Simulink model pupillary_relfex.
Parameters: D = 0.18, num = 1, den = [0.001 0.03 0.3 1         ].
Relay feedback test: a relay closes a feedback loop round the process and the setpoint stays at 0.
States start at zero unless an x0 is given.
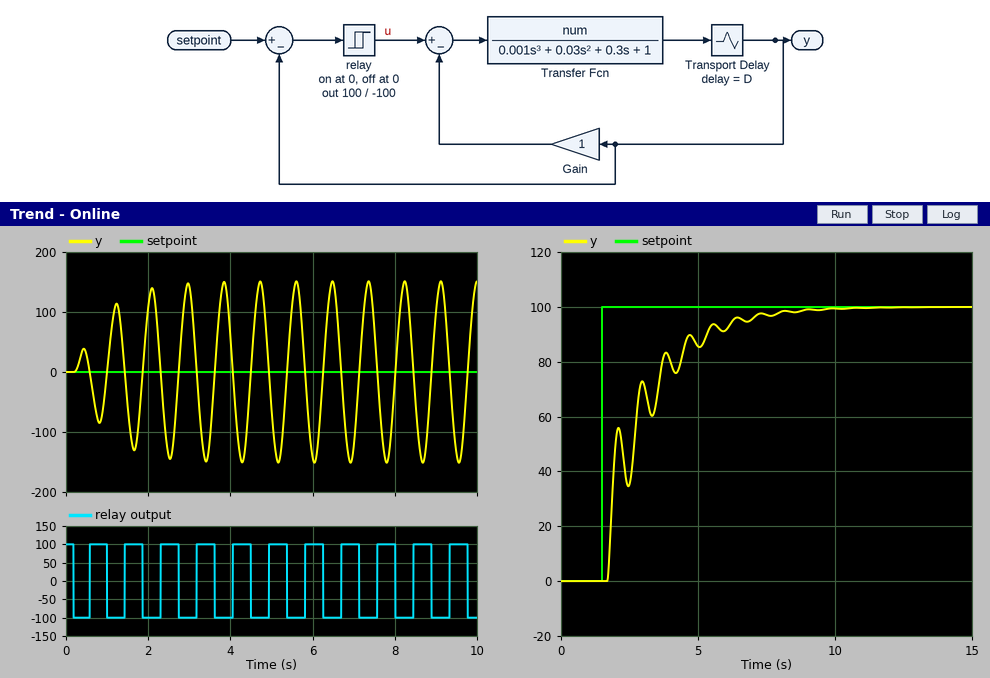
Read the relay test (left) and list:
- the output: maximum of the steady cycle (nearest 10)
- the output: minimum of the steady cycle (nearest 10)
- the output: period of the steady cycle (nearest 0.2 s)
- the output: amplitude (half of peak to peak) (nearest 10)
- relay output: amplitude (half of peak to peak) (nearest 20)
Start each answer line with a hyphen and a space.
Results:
- 150
- -150
- 0.8 s
- 150
- 100
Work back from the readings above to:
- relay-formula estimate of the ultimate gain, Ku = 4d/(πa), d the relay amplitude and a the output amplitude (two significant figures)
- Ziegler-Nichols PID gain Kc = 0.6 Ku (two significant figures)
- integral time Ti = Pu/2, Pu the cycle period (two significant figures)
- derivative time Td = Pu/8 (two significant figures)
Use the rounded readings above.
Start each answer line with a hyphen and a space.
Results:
- 0.85
- 0.51
- 0.40 s
- 0.10 s
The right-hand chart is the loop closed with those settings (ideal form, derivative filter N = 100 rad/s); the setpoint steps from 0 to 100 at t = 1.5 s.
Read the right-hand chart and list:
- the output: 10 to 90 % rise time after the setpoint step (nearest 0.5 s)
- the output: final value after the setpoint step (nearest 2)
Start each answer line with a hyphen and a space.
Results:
- 3.5 s
- 100
